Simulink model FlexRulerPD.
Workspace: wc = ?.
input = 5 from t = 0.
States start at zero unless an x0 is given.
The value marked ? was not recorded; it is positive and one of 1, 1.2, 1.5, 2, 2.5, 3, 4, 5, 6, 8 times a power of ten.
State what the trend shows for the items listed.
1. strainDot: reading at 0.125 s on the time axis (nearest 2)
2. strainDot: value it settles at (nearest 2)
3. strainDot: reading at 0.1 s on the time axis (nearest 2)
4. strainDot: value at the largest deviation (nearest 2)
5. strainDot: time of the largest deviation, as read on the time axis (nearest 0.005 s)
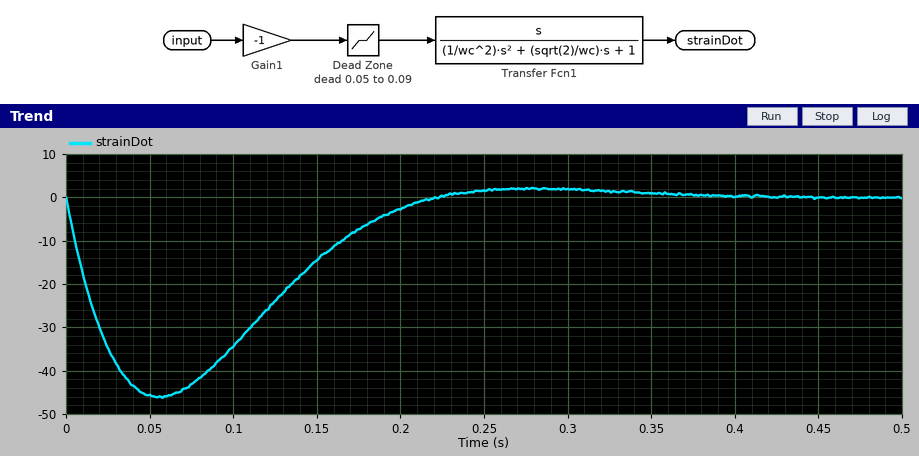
-24
0
-34
-46
0.055 s
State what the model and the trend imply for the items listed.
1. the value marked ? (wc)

20
